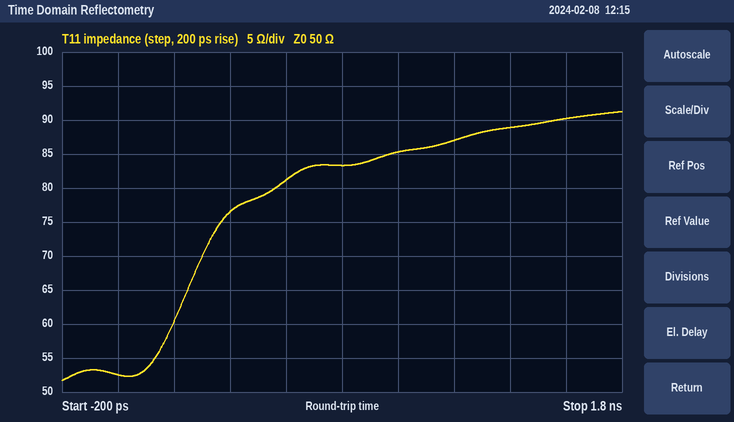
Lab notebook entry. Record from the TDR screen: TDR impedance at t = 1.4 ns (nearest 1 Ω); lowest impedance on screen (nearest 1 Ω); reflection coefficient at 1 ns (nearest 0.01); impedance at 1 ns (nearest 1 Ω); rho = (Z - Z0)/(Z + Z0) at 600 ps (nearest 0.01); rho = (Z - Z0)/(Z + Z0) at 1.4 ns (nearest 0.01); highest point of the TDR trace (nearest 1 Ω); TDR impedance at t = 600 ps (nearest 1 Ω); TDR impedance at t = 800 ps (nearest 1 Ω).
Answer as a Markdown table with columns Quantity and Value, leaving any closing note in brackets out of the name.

| Quantity | Value |
|---|---|
| TDR impedance at t = 1.4 ns | 89 Ω |
| lowest impedance on screen | 52 Ω |
| reflection coefficient at 1 ns | +0.26 |
| impedance at 1 ns | 85 Ω |
| rho = (Z - Z0)/(Z + Z0) at 600 ps | +0.24 |
| rho = (Z - Z0)/(Z + Z0) at 1.4 ns | +0.28 |
| highest point of the TDR trace | 91 Ω |
| TDR impedance at t = 600 ps | 81 Ω |
| TDR impedance at t = 800 ps | 83 Ω |
